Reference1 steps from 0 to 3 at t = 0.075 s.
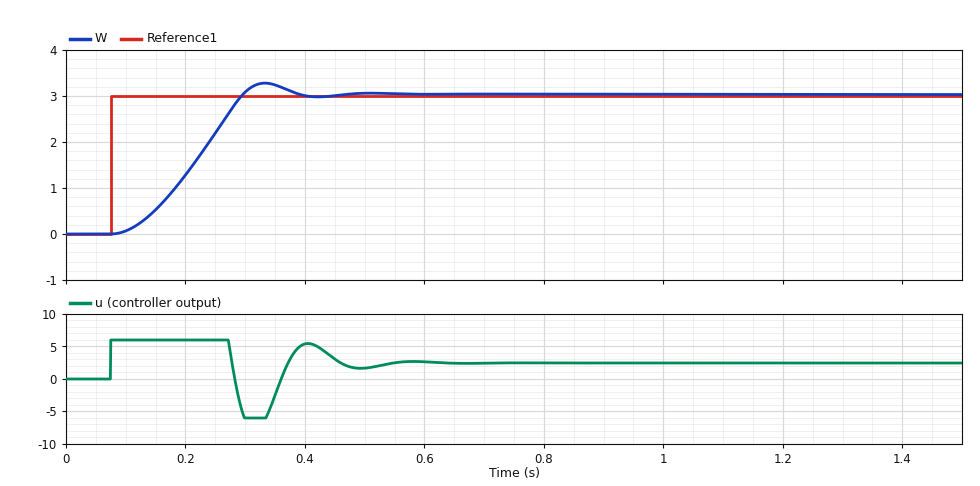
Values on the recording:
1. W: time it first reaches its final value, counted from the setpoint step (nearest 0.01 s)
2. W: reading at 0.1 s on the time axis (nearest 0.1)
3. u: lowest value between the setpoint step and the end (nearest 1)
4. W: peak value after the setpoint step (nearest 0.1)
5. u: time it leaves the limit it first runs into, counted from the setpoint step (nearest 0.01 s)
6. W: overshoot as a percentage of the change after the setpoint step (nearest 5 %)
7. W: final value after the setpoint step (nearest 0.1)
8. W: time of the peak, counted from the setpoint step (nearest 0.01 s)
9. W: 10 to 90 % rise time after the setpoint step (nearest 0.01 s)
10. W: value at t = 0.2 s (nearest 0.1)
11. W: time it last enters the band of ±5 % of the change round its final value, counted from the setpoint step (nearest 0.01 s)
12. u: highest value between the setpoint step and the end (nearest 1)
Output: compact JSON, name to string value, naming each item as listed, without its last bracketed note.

{"W: time it first reaches its final value, counted from the setpoint step": "0.22 s", "W: reading at 0.1 s on the time axis": "0.1", "u: lowest value between the setpoint step and the end": "-6", "W: peak value after the setpoint step": "3.3", "u: time it leaves the limit it first runs into, counted from the setpoint step": "0.20 s", "W: overshoot as a percentage of the change after the setpoint step": "10 %", "W: final value after the setpoint step": "3.0", "W: time of the peak, counted from the setpoint step": "0.26 s", "W: 10 to 90 % rise time after the setpoint step": "0.15 s", "W: value at t = 0.2 s": "1.3", "W: time it last enters the band of ±5 % of the change round its final value, counted from the setpoint step": "0.29 s", "u: highest value between the setpoint step and the end": "6"}
